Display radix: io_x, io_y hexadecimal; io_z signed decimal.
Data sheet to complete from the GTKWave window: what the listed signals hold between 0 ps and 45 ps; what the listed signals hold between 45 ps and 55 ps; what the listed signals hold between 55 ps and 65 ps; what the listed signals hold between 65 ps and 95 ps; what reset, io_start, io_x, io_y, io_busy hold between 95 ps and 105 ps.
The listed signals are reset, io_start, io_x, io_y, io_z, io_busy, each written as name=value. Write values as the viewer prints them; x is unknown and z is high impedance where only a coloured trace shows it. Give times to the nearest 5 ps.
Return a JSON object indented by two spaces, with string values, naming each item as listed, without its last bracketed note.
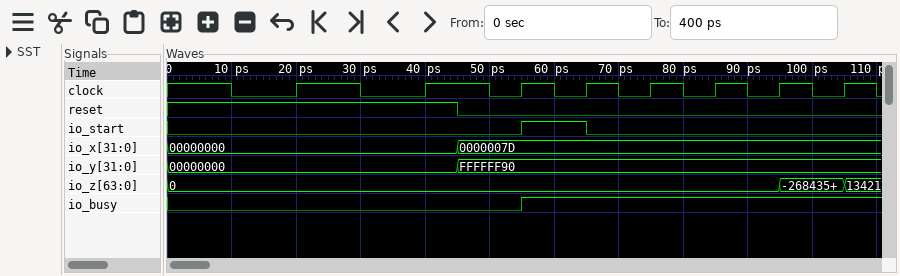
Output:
{
  "what the listed signals hold between 0 ps and 45 ps": "reset=1, io_start=0, io_x=00000000, io_y=00000000, io_z=0, io_busy=0",
  "what the listed signals hold between 45 ps and 55 ps": "reset=0, io_start=0, io_x=0000007D, io_y=FFFFFF90, io_z=0, io_busy=0",
  "what the listed signals hold between 55 ps and 65 ps": "reset=0, io_start=1, io_x=0000007D, io_y=FFFFFF90, io_z=0, io_busy=1",
  "what the listed signals hold between 65 ps and 95 ps": "reset=0, io_start=0, io_x=0000007D, io_y=FFFFFF90, io_z=0, io_busy=1",
  "what reset, io_start, io_x, io_y, io_busy hold between 95 ps and 105 ps": "reset=0, io_start=0, io_x=0000007D, io_y=FFFFFF90, io_busy=1"
}
